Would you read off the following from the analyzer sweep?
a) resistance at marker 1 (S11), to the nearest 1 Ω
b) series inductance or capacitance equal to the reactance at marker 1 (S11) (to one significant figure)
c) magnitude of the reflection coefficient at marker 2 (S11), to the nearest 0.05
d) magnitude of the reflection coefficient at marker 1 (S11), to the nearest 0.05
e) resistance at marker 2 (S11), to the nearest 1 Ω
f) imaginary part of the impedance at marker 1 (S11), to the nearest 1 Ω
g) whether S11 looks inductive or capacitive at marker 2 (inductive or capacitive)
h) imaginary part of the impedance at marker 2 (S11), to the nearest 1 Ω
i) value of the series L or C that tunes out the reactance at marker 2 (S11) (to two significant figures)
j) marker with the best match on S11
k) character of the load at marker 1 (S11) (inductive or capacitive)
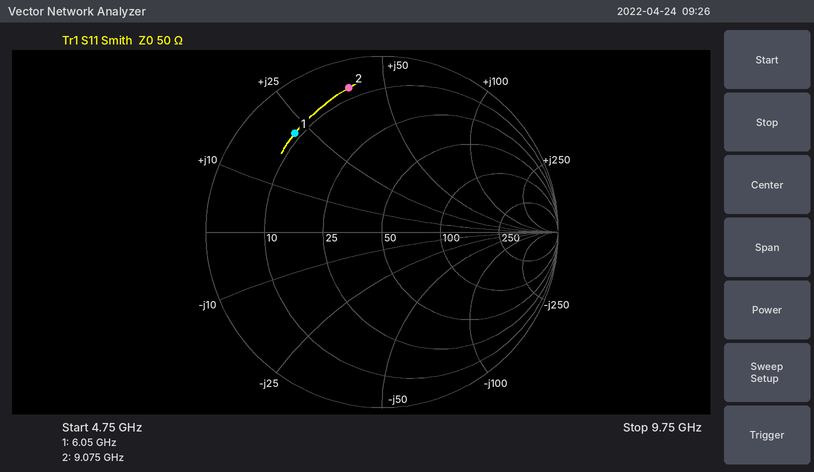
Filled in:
9 Ω
600 pH
0.85
0.75
7 Ω
+22 Ω
inductive
+39 Ω
450 fF
marker 1
inductive
